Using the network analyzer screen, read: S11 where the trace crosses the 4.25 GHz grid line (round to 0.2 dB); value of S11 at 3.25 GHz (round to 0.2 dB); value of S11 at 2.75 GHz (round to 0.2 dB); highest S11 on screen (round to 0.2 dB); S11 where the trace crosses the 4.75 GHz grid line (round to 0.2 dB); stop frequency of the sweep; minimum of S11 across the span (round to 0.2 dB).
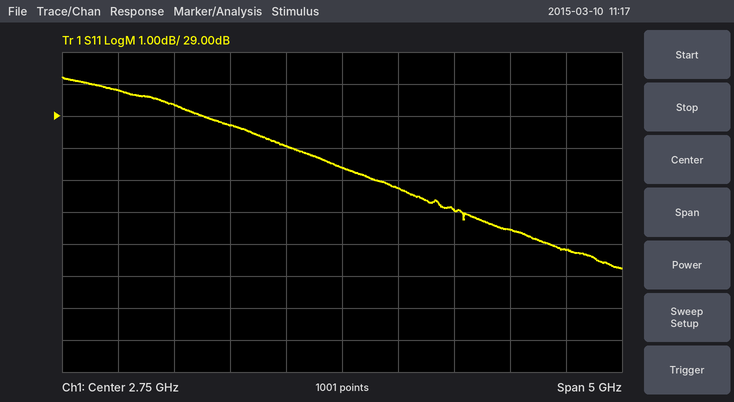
25.4 dB
26.8 dB
27.4 dB
30.2 dB
24.8 dB
5.25 GHz
24.2 dB
